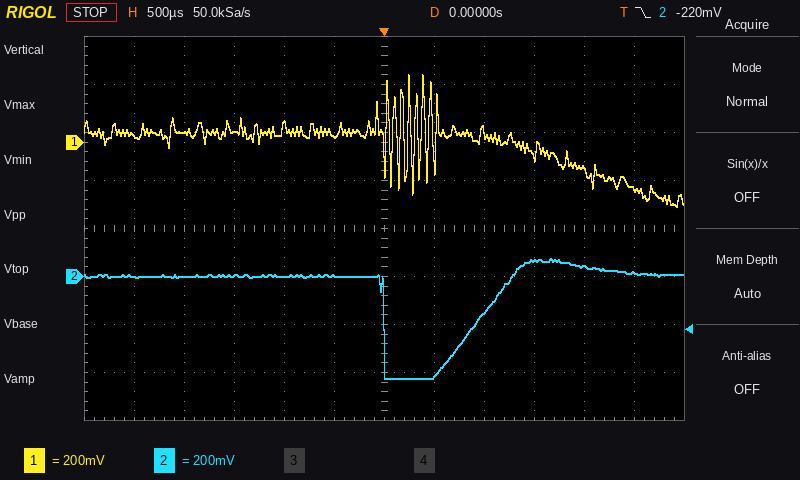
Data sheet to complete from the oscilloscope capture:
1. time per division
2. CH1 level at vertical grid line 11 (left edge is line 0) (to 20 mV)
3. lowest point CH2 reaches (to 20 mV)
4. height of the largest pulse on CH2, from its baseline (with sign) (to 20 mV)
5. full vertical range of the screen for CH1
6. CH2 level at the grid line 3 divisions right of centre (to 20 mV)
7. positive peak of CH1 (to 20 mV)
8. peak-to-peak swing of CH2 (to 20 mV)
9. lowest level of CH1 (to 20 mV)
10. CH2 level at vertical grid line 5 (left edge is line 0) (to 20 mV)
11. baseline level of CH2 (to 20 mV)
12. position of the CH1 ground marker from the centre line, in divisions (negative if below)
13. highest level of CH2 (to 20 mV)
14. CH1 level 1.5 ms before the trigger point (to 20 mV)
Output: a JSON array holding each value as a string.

["500 µs", "-200 mV", "-420 mV", "-420 mV", "1.6 V", "60 mV", "280 mV", "500 mV", "-260 mV", "0 mV", "0 mV", "+1.8 div", "80 mV", "40 mV"]
